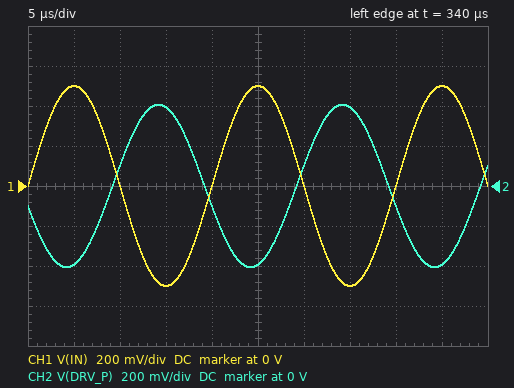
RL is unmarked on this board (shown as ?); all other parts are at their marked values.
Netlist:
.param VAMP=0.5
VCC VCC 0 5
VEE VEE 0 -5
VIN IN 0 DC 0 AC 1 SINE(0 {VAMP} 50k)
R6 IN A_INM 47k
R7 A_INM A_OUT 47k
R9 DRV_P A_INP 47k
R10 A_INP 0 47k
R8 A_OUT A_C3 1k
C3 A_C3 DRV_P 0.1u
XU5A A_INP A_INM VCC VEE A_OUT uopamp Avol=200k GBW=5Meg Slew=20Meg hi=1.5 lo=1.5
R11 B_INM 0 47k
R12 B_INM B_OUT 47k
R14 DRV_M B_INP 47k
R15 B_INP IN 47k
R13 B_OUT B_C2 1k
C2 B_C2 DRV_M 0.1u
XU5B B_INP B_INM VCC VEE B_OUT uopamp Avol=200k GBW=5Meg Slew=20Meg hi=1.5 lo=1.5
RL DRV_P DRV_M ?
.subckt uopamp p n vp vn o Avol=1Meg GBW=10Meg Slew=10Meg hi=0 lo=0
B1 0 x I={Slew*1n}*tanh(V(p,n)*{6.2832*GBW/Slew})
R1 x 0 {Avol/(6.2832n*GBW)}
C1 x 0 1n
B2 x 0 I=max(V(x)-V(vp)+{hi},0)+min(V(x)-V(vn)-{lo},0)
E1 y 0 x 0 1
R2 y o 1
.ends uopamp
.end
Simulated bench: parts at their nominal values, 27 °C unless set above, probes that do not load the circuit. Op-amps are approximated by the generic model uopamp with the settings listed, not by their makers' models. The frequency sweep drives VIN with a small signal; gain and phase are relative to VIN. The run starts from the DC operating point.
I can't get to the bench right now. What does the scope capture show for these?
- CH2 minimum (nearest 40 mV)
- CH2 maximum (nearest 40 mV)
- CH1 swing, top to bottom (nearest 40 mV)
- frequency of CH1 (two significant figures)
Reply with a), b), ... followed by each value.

a) -400 mV
b) 400 mV
c) 1.00 V
d) 50 kHz
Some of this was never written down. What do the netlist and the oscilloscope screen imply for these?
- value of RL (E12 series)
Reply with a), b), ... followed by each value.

a) 1.8 kΩ
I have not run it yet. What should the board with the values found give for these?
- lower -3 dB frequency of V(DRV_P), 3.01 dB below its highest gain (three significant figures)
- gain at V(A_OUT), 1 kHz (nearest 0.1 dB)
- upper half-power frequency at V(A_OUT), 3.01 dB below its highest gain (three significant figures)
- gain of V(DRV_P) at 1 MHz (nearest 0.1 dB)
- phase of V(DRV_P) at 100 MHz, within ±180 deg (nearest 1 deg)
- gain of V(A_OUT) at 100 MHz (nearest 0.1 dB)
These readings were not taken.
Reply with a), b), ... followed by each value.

a) 17.0 kHz
b) -1.4 dB
c) 1.35 MHz
d) -3.1 dB
e) 77 deg
f) -32.1 dB
